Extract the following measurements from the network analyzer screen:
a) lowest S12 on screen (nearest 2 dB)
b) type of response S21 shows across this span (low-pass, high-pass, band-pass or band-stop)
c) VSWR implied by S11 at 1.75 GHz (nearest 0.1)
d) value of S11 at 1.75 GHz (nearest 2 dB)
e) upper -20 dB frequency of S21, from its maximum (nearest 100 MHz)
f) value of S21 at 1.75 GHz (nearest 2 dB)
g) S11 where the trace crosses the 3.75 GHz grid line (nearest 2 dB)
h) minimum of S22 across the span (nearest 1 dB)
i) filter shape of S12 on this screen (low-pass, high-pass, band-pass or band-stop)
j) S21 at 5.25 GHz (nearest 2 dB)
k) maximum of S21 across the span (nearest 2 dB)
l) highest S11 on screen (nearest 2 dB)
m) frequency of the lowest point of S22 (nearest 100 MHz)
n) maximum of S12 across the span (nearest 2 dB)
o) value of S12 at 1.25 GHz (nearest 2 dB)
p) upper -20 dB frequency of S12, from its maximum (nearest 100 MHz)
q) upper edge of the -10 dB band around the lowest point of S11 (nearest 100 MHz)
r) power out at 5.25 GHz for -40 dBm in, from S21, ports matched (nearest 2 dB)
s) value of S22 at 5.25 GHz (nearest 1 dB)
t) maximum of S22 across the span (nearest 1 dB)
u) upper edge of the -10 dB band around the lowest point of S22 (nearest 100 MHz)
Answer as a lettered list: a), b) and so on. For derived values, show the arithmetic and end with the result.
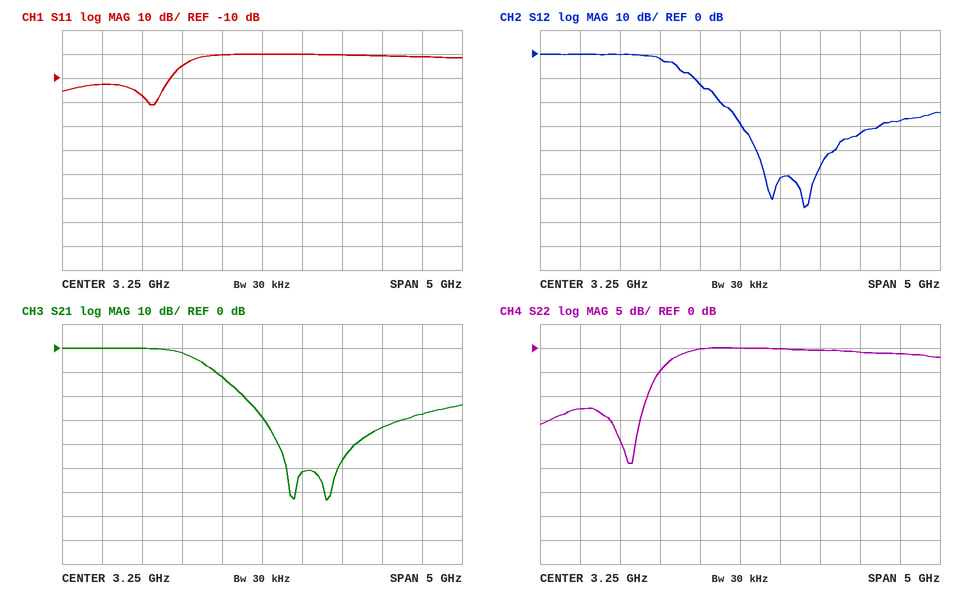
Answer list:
a) -64 dB
b) low-pass
c) |Γ| = 10^(-18/20) = 0.1259; VSWR = (1 + 0.1259)/(1 − 0.1259) ≈ 1.3
d) -18 dB
e) 3.0 GHz
f) 0 dB
g) 0 dB
h) -24 dB
i) low-pass
j) -28 dB
k) 0 dB
l) 0 dB
m) 1.9 GHz
n) 0 dB
o) 0 dB
p) 3.0 GHz
q) 2.1 GHz
r) -40 dBm + (-28 dB) = -68 dBm
s) -1 dB
t) 0 dB
u) 2.1 GHz
